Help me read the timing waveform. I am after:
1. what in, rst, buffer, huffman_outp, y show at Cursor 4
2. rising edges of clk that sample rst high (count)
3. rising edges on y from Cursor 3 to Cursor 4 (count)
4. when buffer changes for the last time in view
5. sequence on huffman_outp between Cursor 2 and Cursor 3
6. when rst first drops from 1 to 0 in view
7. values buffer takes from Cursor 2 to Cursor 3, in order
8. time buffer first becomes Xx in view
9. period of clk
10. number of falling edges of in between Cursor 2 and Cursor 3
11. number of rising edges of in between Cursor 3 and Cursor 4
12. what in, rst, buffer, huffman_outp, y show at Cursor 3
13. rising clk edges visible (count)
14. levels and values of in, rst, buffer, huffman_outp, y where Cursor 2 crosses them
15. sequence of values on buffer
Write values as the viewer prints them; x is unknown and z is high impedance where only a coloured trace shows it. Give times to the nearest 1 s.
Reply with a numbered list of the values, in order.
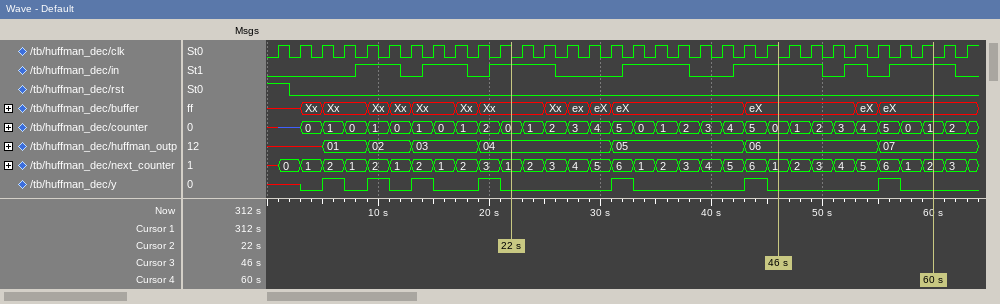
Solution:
1. in=1, rst=0, buffer=eX, huffman_outp=07, y=0
2. 1
3. 1
4. 55 s
5. 04, 05, 06
6. 2 s
7. Xx, Xx, ex, eX, eX, eX
8. 3 s
9. 2 s
10. 2
11. 2
12. in=1, rst=0, buffer=eX, huffman_outp=06, y=0
13. 32
14. in=1, rst=0, buffer=Xx, huffman_outp=04, y=0
15. x, Xx, Xx, Xx, Xx, Xx, Xx, Xx, Xx, ex, eX, eX, eX, eX, eX
